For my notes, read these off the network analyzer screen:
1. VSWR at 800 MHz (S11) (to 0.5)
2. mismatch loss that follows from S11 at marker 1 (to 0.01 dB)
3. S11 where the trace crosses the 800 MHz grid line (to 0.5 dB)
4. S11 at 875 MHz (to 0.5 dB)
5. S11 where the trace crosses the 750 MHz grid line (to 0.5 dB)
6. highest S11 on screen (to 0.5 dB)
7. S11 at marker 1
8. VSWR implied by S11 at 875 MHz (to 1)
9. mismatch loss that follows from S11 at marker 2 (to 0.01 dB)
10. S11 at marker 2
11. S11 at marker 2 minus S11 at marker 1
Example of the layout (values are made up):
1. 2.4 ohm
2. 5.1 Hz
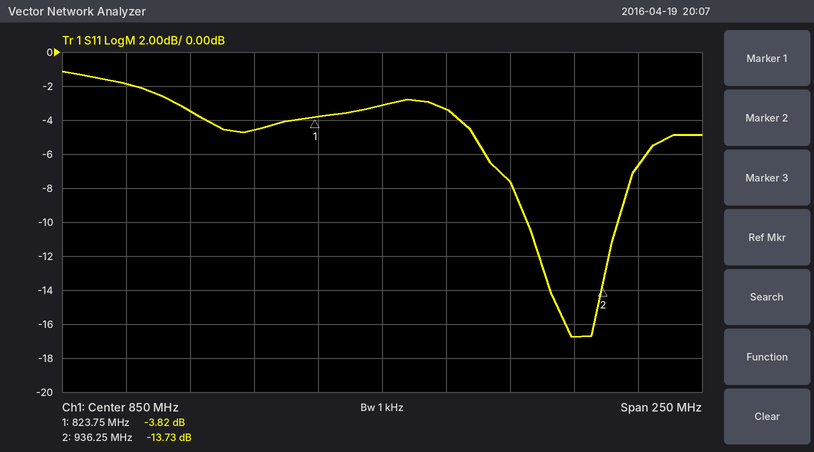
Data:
1. 4.0
2. 2.33 dB
3. -4.5 dB
4. -3.5 dB
5. -2.0 dB
6. -1.0 dB
7. -3.82 dB
8. 5
9. 0.19 dB
10. -13.73 dB
11. -9.91 dB
